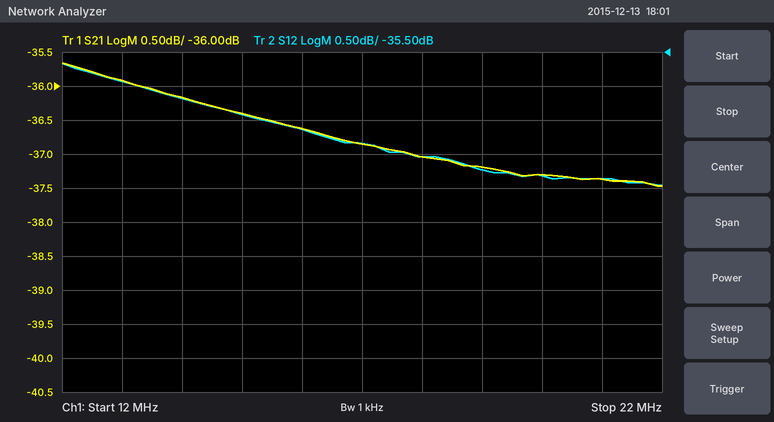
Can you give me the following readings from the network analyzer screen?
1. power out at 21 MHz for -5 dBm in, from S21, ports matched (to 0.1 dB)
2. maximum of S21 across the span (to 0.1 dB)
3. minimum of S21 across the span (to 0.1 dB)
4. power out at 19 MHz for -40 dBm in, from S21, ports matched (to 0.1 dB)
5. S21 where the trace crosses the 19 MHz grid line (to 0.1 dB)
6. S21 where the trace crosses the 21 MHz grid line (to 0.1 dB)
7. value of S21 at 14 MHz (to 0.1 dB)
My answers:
-42.4 dBm
-35.7 dB
-37.5 dB
-77.2 dBm
-37.2 dB
-37.4 dB
-36.2 dB
